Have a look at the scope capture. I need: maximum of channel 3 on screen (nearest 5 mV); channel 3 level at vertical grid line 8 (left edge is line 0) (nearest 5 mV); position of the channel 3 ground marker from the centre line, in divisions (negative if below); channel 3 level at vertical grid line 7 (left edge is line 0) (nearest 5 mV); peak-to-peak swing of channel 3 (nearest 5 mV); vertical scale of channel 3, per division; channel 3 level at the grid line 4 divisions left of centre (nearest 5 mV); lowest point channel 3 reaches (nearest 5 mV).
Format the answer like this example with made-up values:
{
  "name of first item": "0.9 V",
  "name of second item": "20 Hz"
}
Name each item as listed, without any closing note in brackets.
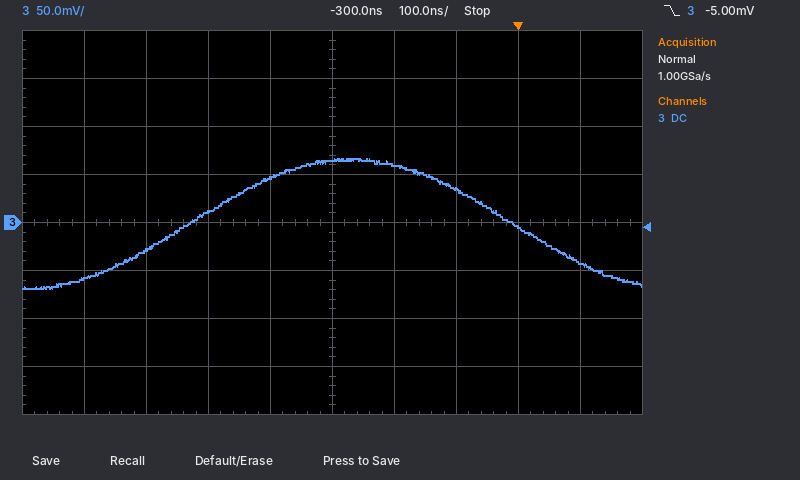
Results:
{
  "maximum of channel 3 on screen": "65 mV",
  "channel 3 level at vertical grid line 8 (left edge is line 0)": "-5 mV",
  "position of the channel 3 ground marker from the centre line, in divisions": "0.0 div",
  "channel 3 level at vertical grid line 7 (left edge is line 0)": "35 mV",
  "peak-to-peak swing of channel 3": "135 mV",
  "vertical scale of channel 3, per division": "50 mV",
  "channel 3 level at the grid line 4 divisions left of centre": "-60 mV",
  "lowest point channel 3 reaches": "-70 mV"
}
